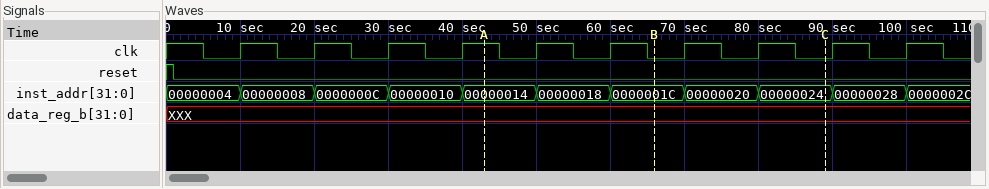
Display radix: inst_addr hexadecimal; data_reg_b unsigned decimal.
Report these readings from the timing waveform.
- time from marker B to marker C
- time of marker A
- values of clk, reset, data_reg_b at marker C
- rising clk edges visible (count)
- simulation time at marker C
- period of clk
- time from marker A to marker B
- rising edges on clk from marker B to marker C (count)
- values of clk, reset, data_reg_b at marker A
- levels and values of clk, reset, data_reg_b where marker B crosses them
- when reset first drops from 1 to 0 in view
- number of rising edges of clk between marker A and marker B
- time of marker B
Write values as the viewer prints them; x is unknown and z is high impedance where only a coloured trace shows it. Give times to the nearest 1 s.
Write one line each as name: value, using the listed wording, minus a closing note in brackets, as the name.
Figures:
time from marker B to marker C: 23 s
time of marker A: 43 s
values of clk, reset, data_reg_b at marker C: clk=0, reset=0, data_reg_b=XXX
rising clk edges visible: 10
simulation time at marker C: 89 s
period of clk: 10 s
time from marker A to marker B: 23 s
rising edges on clk from marker B to marker C: 2
values of clk, reset, data_reg_b at marker A: clk=1, reset=0, data_reg_b=XXX
levels and values of clk, reset, data_reg_b where marker B crosses them: clk=0, reset=0, data_reg_b=XXX
when reset first drops from 1 to 0 in view: 1 s
number of rising edges of clk between marker A and marker B: 2
time of marker B: 66 s
